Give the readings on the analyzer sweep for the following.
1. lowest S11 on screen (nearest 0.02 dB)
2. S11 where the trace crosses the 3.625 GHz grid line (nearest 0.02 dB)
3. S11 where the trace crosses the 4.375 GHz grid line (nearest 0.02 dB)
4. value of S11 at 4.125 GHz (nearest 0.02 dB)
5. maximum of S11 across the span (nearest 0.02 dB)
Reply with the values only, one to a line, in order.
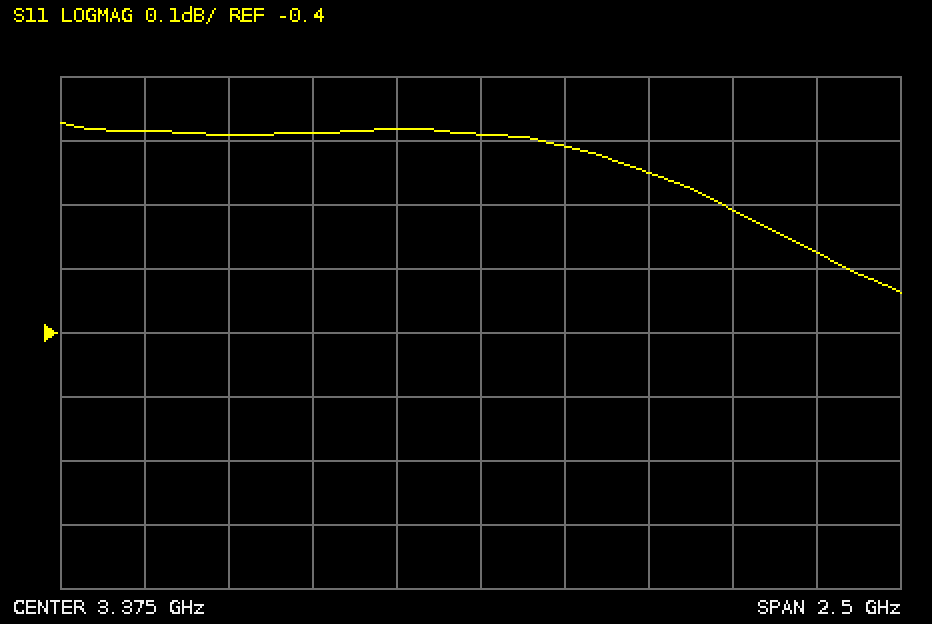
-0.34 dB
-0.10 dB
-0.28 dB
-0.20 dB
-0.08 dB
